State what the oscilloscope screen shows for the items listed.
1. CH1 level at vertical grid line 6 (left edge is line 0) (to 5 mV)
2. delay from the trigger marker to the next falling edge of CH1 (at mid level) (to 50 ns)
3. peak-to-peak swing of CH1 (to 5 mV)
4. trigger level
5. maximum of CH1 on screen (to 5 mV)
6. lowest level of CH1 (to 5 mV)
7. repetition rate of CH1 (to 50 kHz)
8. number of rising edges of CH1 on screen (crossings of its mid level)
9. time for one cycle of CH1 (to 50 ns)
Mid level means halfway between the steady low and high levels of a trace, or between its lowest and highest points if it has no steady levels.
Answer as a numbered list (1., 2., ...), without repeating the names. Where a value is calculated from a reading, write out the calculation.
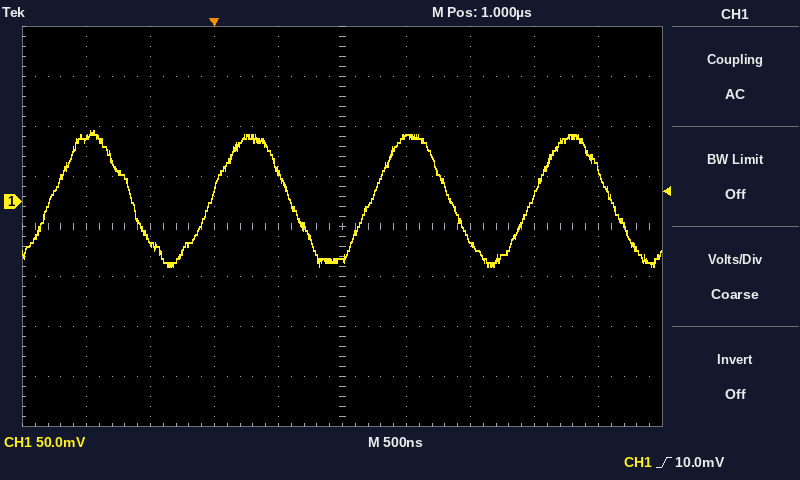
1. 65 mV
2. 600 ns
3. 70 mV − (-65 mV) = 135 mV
4. 10.0 mV
5. 70 mV
6. -65 mV
7. 1 / 1.25 µs ≈ 800 kHz
8. 4
9. 1.25 µs
